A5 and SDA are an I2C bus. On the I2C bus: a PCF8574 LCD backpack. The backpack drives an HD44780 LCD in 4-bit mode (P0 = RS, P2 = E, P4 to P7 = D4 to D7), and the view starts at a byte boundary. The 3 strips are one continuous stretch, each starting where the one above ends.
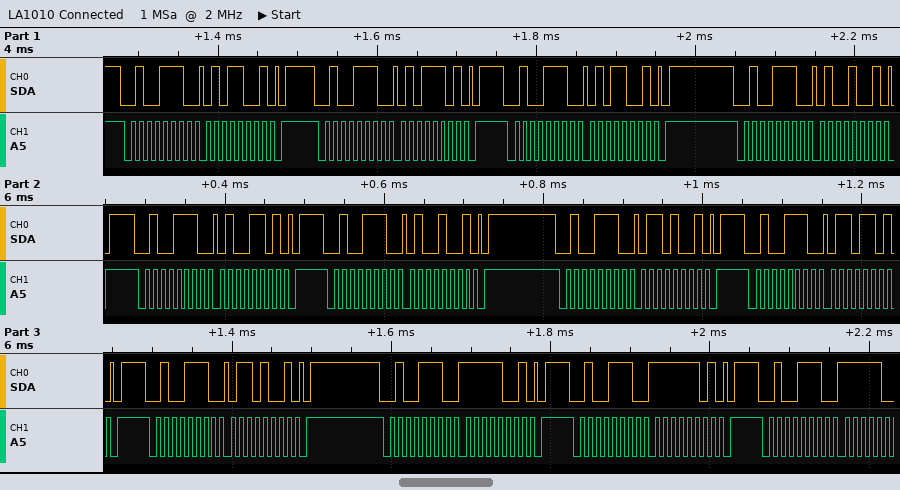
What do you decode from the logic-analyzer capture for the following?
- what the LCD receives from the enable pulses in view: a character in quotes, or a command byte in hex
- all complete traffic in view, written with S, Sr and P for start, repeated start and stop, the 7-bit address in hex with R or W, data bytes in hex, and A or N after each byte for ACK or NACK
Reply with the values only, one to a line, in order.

'T'
S 27W A 59 A P S 27W A 5D A P S 27W A 59 A P S 27W A 49 A P S 27W A 4D A P S 27W A 49 A P S 27W A 69 A P S 27W A 6D A P S 27W A 69 A P S 27W A F9 A P S 27W A FD A P S 27W A
